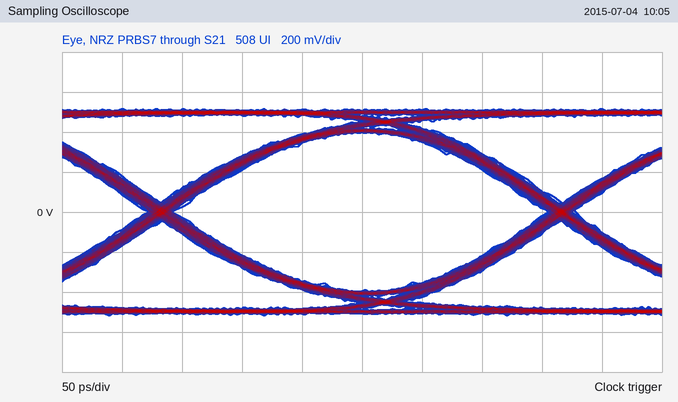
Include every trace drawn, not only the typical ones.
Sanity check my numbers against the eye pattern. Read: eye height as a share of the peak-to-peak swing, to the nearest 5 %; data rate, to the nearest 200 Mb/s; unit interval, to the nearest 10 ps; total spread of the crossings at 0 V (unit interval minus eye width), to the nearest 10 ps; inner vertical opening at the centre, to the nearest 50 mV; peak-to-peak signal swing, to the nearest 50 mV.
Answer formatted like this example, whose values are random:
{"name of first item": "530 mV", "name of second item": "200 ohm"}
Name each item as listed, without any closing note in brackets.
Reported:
{"eye height as a share of the peak-to-peak swing, to the nearest 5 %": "75 %", "data rate, to the nearest 200 Mb/s": "3.0 Gb/s", "unit interval, to the nearest 10 ps": "330 ps", "total spread of the crossings at 0 V (unit interval minus eye width), to the nearest 10 ps": "20 ps", "inner vertical opening at the centre, to the nearest 50 mV": "800 mV", "peak-to-peak signal swing, to the nearest 50 mV": "1.05 V"}
